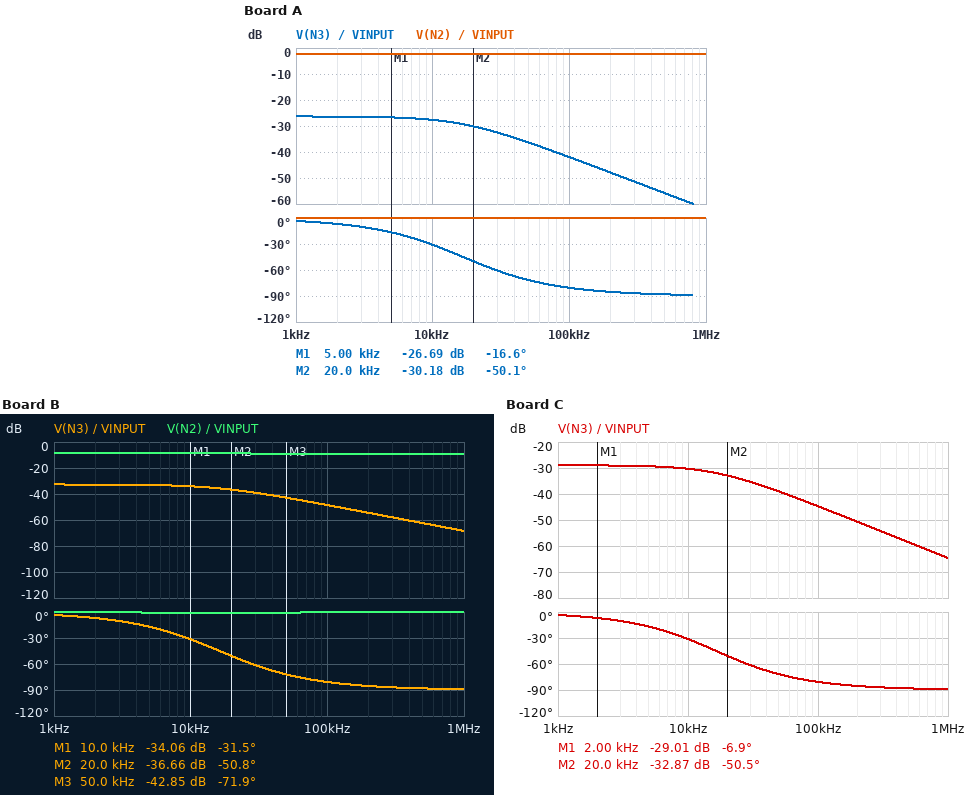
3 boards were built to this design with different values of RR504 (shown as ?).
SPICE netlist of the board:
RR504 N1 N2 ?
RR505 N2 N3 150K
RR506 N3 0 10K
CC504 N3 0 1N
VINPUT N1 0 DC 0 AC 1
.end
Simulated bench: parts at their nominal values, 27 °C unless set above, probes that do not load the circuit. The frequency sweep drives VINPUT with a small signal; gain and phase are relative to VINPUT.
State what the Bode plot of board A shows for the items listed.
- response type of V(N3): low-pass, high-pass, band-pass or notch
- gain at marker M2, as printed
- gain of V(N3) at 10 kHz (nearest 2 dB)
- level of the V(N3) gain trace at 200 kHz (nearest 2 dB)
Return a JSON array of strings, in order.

["low-pass", "-30.18 dB", "-28 dB", "-48 dB"]
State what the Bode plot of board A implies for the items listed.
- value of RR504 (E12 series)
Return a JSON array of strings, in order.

["47 kΩ"]
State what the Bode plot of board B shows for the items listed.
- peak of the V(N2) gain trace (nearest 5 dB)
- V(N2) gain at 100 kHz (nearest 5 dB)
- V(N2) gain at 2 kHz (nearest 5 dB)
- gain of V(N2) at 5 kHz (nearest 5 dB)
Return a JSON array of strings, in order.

["-10 dB", "-10 dB", "-10 dB", "-10 dB"]
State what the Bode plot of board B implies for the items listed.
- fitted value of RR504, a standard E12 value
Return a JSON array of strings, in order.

["270 kΩ"]
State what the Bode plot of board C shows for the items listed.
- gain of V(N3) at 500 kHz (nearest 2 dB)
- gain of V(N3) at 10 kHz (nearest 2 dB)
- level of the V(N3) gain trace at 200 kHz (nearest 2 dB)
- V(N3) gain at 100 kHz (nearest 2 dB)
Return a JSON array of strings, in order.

["-58 dB", "-30 dB", "-50 dB", "-44 dB"]
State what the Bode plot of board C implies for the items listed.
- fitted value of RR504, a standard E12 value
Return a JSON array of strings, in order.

["120 kΩ"]
